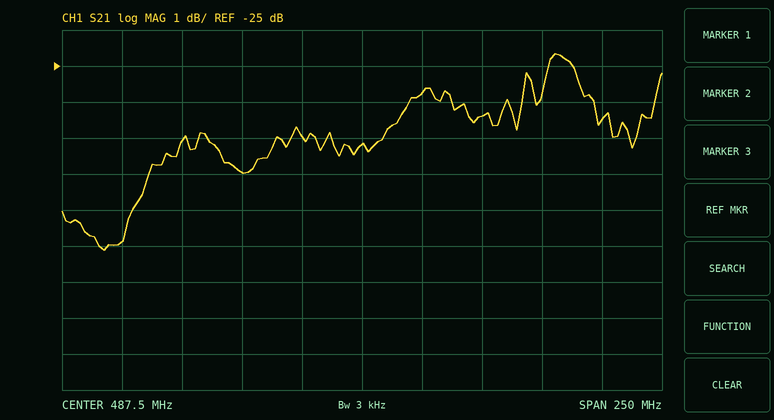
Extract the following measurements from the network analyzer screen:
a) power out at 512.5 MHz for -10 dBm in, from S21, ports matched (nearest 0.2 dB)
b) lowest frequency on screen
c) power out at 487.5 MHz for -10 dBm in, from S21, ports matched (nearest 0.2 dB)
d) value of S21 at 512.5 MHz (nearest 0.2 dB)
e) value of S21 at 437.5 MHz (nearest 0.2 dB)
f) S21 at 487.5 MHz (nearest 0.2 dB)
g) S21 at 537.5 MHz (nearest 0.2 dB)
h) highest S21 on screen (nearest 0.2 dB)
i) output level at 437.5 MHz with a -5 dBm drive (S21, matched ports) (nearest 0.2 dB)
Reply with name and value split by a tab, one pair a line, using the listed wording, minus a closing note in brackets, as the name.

power out at 512.5 MHz for -10 dBm in, from S21, ports matched	-35.8 dBm
lowest frequency on screen	362.5 MHz
power out at 487.5 MHz for -10 dBm in, from S21, ports matched	-37.2 dBm
value of S21 at 512.5 MHz	-25.8 dB
value of S21 at 437.5 MHz	-28.0 dB
S21 at 487.5 MHz	-27.2 dB
S21 at 537.5 MHz	-26.4 dB
highest S21 on screen	-24.6 dB
output level at 437.5 MHz with a -5 dBm drive (S21, matched ports)	-33.0 dBm
